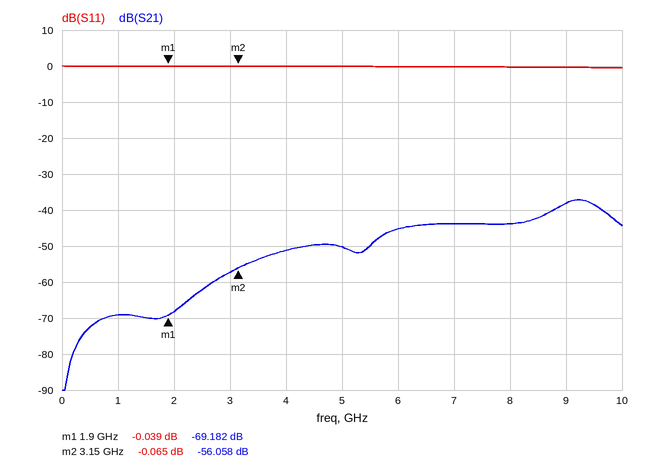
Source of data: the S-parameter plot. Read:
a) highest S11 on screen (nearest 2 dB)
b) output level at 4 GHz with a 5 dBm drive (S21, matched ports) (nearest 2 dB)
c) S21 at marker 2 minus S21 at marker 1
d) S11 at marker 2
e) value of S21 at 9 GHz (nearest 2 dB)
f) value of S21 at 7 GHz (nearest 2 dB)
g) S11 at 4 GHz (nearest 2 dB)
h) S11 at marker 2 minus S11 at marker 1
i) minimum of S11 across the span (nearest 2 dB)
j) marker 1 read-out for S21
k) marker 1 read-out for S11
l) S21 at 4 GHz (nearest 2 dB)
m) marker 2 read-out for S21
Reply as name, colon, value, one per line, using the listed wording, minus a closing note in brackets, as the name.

highest S11 on screen: 0 dB
output level at 4 GHz with a 5 dBm drive (S21, matched ports): -46 dBm
S21 at marker 2 minus S21 at marker 1: 13.124 dB
S11 at marker 2: -0.065 dB
value of S21 at 9 GHz: -38 dB
value of S21 at 7 GHz: -44 dB
S11 at 4 GHz: 0 dB
S11 at marker 2 minus S11 at marker 1: -0.026 dB
minimum of S11 across the span: 0 dB
marker 1 read-out for S21: -69.182 dB
marker 1 read-out for S11: -0.039 dB
S21 at 4 GHz: -52 dB
marker 2 read-out for S21: -56.058 dB
